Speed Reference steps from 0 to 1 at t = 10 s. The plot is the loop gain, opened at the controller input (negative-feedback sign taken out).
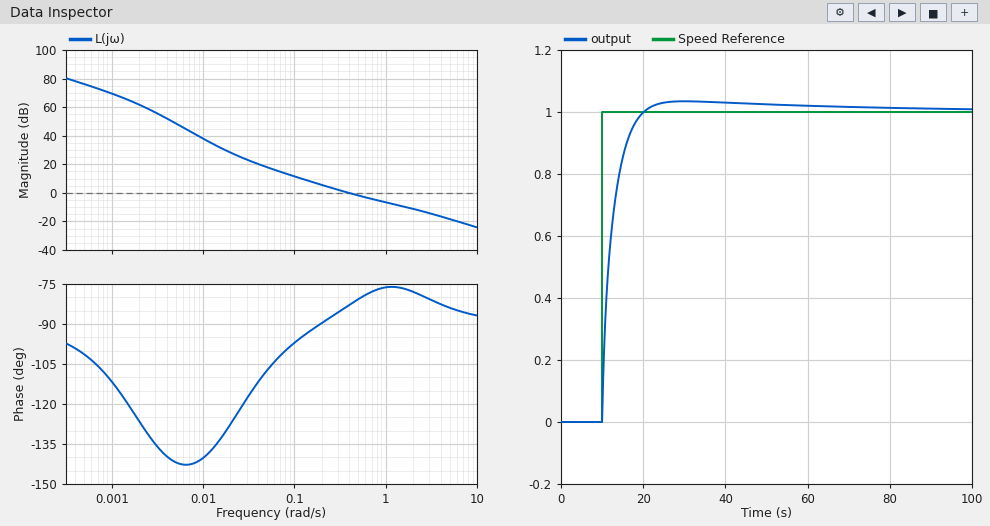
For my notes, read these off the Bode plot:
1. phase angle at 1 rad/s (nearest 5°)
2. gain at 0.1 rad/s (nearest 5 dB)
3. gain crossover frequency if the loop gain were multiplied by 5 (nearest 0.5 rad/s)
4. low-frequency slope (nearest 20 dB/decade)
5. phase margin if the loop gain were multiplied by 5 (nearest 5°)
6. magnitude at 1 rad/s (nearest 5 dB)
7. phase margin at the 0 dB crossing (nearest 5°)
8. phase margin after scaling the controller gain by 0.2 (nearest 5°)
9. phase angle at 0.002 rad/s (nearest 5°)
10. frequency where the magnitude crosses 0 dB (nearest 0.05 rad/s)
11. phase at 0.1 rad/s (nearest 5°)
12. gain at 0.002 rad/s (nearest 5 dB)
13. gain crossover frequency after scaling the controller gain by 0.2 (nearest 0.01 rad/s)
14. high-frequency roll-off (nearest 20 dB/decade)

-75°
10 dB
3.0 rad/s
-20 dB/decade
100°
-5 dB
95°
80°
-125°
0.40 rad/s
-95°
60 dB
0.08 rad/s
-20 dB/decade
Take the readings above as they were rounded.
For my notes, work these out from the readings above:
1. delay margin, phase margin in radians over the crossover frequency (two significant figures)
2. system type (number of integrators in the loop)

4.1 s
1
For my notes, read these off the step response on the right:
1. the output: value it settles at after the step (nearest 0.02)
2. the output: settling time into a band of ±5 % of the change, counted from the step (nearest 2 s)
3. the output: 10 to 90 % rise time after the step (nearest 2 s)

1.00
8 s
6 s
